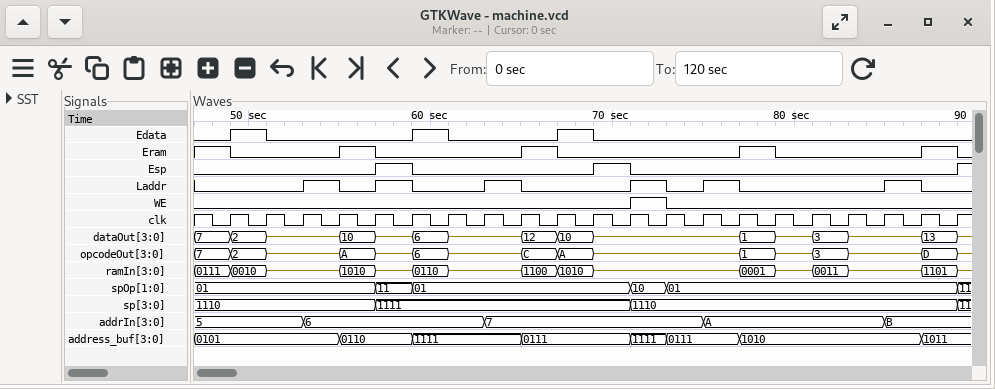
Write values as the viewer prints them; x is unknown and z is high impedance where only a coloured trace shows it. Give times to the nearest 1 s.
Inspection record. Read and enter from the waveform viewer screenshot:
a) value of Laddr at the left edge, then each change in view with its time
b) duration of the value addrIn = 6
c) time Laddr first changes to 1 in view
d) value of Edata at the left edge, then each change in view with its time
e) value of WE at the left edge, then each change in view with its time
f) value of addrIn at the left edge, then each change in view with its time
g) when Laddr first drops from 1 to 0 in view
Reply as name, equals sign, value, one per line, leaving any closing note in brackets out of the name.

value of Laddr at the left edge, then each change in view with its time = 0, 1 at 53 s, 0 at 55 s, 1 at 57 s, 0 at 59 s, 1 at 63 s, 0 at 65 s, 1 at 71 s, 0 at 73 s, 1 at 75 s, 0 at 77 s, 1 at 85 s, 0 at 87 s
duration of the value addrIn = 6 = 10 s
time Laddr first changes to 1 in view = 53 s
value of Edata at the left edge, then each change in view with its time = 0, 1 at 49 s, 0 at 51 s, 1 at 59 s, 0 at 61 s, 1 at 67 s, 0 at 69 s
value of WE at the left edge, then each change in view with its time = 0, 1 at 71 s, 0 at 73 s
value of addrIn at the left edge, then each change in view with its time = 5, 6 at 53 s, 7 at 63 s, A at 75 s, B at 85 s
when Laddr first drops from 1 to 0 in view = 55 s
